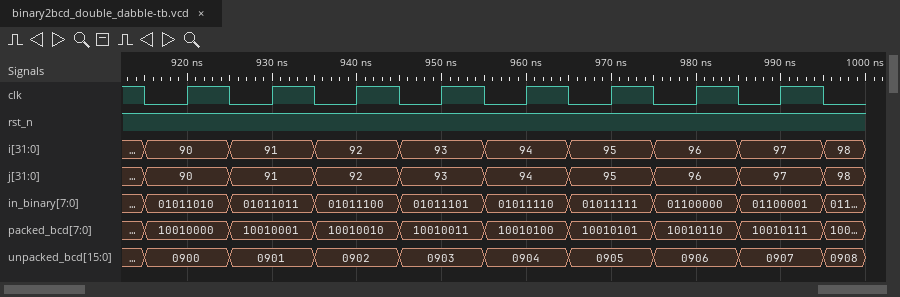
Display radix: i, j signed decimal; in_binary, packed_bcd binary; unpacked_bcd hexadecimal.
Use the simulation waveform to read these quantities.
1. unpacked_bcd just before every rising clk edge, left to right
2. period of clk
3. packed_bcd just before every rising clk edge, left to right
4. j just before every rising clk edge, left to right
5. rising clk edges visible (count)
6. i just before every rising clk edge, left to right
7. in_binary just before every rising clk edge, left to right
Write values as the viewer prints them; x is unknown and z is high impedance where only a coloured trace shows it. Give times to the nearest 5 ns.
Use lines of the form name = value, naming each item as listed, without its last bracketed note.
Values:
unpacked_bcd just before every rising clk edge, left to right = 0900, 0901, 0902, 0903, 0904, 0905, 0906, 0907
period of clk = 10 ns
packed_bcd just before every rising clk edge, left to right = 10010000, 10010001, 10010010, 10010011, 10010100, 10010101, 10010110, 10010111
j just before every rising clk edge, left to right = 90, 91, 92, 93, 94, 95, 96, 97
rising clk edges visible = 8
i just before every rising clk edge, left to right = 90, 91, 92, 93, 94, 95, 96, 97
in_binary just before every rising clk edge, left to right = 01011010, 01011011, 01011100, 01011101, 01011110, 01011111, 01100000, 01100001
